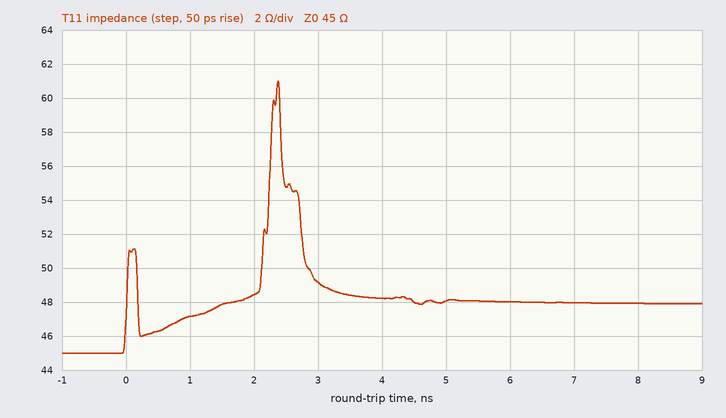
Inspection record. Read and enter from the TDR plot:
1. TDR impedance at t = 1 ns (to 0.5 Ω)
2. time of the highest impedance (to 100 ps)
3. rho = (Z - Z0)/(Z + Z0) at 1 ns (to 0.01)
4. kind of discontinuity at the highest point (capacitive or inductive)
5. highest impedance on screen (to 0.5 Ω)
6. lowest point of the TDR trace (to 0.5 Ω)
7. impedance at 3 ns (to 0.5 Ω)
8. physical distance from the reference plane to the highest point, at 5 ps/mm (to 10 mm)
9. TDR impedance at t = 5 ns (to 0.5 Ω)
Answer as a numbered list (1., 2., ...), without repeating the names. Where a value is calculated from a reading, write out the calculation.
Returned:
1. 47.0 Ω
2. 2.4 ns
3. (47 − 45)/(47 + 45) ≈ +0.02
4. inductive
5. 61.0 Ω
6. 45.0 Ω
7. 49.0 Ω
8. 2.4 ns / 2 / 5 ps/mm ≈ 240 mm
9. 48.0 Ω
